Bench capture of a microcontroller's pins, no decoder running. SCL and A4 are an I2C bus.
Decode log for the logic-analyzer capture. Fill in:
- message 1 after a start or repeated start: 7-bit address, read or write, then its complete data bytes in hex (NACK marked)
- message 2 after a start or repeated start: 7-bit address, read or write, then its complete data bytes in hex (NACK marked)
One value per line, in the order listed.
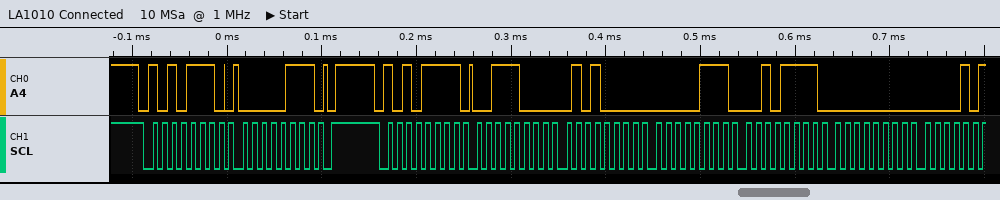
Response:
0x57 write: 07
0x57 read: 38 50 07 2F 00
